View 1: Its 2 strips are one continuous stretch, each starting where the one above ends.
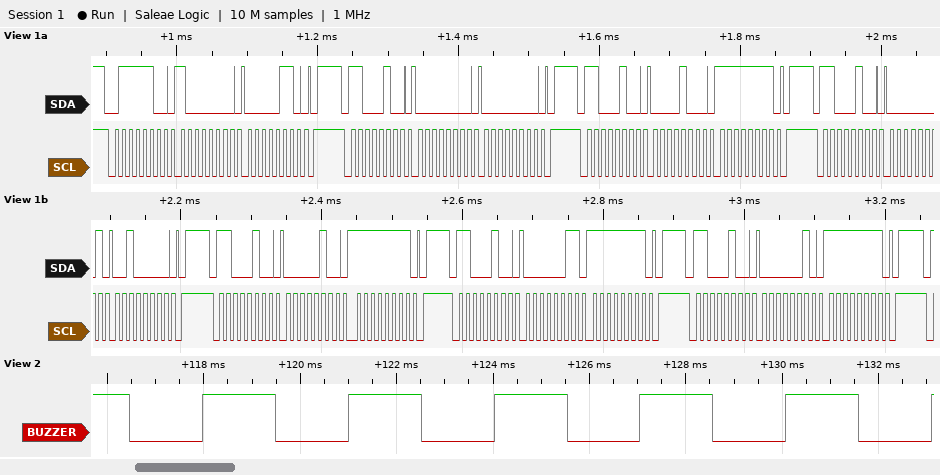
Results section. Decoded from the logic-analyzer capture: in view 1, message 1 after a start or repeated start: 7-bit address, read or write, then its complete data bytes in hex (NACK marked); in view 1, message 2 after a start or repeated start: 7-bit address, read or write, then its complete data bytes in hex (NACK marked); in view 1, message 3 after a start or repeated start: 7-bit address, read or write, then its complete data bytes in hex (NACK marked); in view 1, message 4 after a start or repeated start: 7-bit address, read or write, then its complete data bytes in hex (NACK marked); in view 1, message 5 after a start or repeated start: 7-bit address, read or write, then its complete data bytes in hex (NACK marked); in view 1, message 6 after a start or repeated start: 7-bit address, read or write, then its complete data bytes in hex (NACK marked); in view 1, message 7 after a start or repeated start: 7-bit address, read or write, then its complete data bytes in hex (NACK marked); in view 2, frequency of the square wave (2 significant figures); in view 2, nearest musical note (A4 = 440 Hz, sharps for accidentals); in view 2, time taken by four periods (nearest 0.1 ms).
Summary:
0x3E write: 80 06
0x62 write: 00 00
0x62 write: 08 FF
0x62 write: 01 20
0x62 write: 04 FF
0x62 write: 03 FF
0x62 write: 02 FF
330 Hz
E4
12.1 ms
